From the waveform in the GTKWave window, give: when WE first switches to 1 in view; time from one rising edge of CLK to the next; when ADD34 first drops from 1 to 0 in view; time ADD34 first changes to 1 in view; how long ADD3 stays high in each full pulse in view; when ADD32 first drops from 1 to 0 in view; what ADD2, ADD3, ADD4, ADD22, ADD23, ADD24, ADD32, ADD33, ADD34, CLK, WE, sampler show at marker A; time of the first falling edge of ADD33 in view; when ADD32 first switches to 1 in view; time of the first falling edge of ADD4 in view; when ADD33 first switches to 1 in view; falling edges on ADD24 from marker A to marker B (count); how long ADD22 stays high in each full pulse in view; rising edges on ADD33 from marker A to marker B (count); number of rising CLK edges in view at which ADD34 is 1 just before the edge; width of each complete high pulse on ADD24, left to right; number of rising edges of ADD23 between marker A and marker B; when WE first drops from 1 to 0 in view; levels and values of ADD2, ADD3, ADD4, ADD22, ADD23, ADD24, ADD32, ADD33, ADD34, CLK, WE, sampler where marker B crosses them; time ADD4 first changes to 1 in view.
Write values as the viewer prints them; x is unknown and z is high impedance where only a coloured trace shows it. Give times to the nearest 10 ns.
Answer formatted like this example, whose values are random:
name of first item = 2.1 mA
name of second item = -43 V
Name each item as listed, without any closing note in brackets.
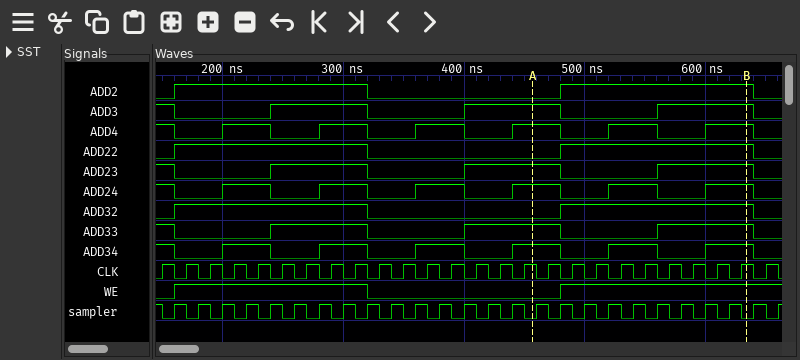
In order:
when WE first switches to 1 in view = 160 ns
time from one rising edge of CLK to the next = 20 ns
when ADD34 first drops from 1 to 0 in view = 160 ns
time ADD34 first changes to 1 in view = 200 ns
how long ADD3 stays high in each full pulse in view = 80 ns, 80 ns, 80 ns
when ADD32 first drops from 1 to 0 in view = 320 ns
what ADD2, ADD3, ADD4, ADD22, ADD23, ADD24, ADD32, ADD33, ADD34, CLK, WE, sampler show at marker A = ADD2=0, ADD3=1, ADD4=1, ADD22=0, ADD23=1, ADD24=1, ADD32=0, ADD33=1, ADD34=1, CLK=1, WE=0, sampler=0
time of the first falling edge of ADD33 in view = 160 ns
when ADD32 first switches to 1 in view = 160 ns
time of the first falling edge of ADD4 in view = 160 ns
when ADD33 first switches to 1 in view = 240 ns
falling edges on ADD24 from marker A to marker B = 2
how long ADD22 stays high in each full pulse in view = 160 ns, 160 ns
rising edges on ADD33 from marker A to marker B = 1
number of rising CLK edges in view at which ADD34 is 1 just before the edge = 13
width of each complete high pulse on ADD24, left to right = 40 ns, 40 ns, 40 ns, 40 ns, 40 ns, 40 ns
number of rising edges of ADD23 between marker A and marker B = 1
when WE first drops from 1 to 0 in view = 320 ns
levels and values of ADD2, ADD3, ADD4, ADD22, ADD23, ADD24, ADD32, ADD33, ADD34, CLK, WE, sampler where marker B crosses them = ADD2=1, ADD3=1, ADD4=1, ADD22=1, ADD23=1, ADD24=1, ADD32=1, ADD33=1, ADD34=1, CLK=1, WE=1, sampler=0
time ADD4 first changes to 1 in view = 200 ns
